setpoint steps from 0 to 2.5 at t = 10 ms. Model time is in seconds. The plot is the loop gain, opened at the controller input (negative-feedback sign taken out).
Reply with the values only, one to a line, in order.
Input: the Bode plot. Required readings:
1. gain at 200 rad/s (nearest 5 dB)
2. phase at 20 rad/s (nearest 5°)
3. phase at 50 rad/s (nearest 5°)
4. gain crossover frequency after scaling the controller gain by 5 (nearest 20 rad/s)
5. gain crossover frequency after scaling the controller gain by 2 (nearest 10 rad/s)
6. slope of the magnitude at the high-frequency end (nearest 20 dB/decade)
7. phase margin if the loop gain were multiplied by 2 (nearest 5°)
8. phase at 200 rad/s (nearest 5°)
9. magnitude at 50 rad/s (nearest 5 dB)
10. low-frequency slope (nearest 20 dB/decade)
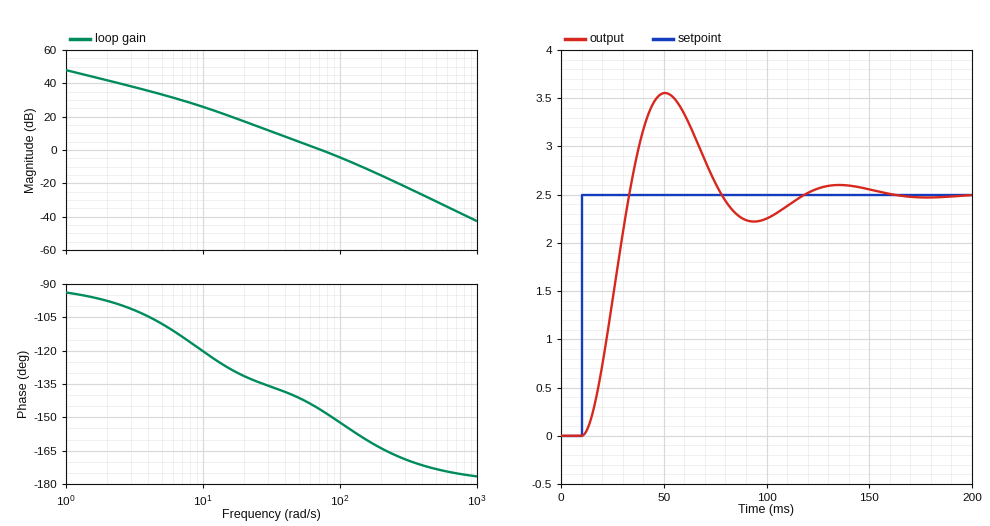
-15 dB
-130°
-140°
180 rad/s
110 rad/s
-40 dB/decade
25°
-165°
5 dB
-20 dB/decade
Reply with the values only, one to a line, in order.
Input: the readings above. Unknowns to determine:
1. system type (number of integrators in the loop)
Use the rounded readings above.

1
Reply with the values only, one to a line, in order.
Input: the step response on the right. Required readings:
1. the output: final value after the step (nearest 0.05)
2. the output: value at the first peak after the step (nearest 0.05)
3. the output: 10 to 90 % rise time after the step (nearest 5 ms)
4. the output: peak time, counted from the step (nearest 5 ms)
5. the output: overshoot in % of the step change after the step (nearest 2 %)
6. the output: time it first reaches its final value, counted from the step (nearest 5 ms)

2.50
3.55
15 ms
40 ms
42 %
25 ms
